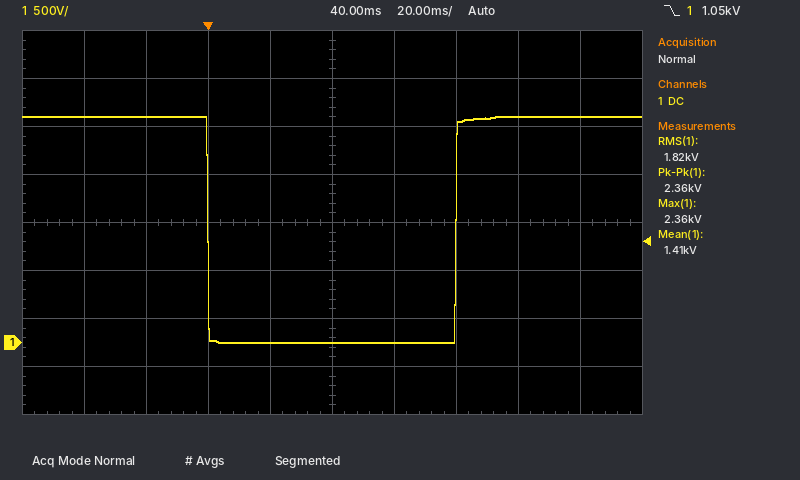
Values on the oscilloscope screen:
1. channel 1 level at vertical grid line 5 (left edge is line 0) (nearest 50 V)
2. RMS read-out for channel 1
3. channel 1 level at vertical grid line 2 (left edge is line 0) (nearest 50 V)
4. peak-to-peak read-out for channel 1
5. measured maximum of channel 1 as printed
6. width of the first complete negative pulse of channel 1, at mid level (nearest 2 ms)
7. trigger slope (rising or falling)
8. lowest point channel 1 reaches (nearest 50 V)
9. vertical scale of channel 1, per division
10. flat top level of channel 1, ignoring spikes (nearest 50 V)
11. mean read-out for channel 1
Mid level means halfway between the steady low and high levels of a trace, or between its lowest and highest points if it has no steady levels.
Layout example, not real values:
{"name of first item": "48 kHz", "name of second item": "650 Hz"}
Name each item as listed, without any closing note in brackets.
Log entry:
{"channel 1 level at vertical grid line 5 (left edge is line 0)": "0 V", "RMS read-out for channel 1": "1.82 kV", "channel 1 level at vertical grid line 2 (left edge is line 0)": "2.35 kV", "peak-to-peak read-out for channel 1": "2.36 kV", "measured maximum of channel 1 as printed": "2.36 kV", "width of the first complete negative pulse of channel 1, at mid level": "80 ms", "trigger slope": "falling", "lowest point channel 1 reaches": "0 V", "vertical scale of channel 1, per division": "500 V", "flat top level of channel 1, ignoring spikes": "2.35 kV", "mean read-out for channel 1": "1.41 kV"}
